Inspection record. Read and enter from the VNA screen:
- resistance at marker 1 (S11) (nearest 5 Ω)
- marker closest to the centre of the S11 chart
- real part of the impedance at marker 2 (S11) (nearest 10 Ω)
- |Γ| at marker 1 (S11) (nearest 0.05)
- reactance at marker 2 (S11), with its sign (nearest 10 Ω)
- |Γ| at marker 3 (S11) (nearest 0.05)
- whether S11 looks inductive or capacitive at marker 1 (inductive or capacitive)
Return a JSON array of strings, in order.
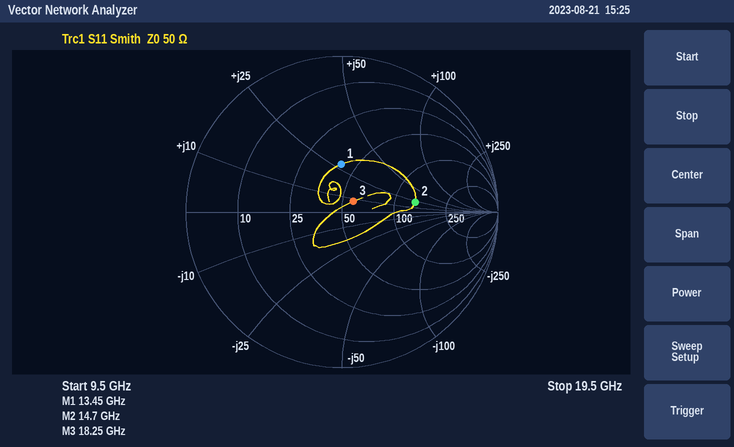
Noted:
["40 Ω", "marker 3", "140 Ω", "0.30", "+20 Ω", "0.10", "inductive"]
